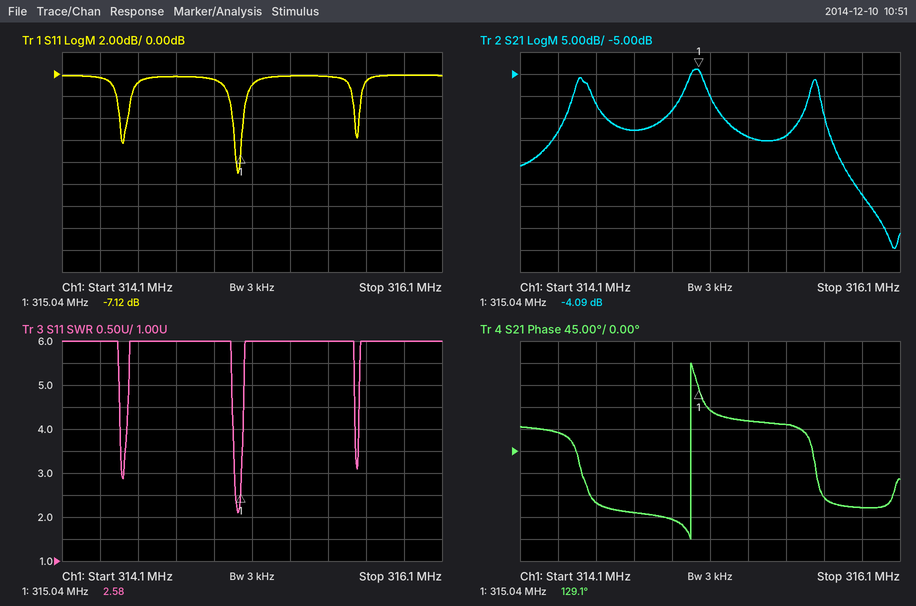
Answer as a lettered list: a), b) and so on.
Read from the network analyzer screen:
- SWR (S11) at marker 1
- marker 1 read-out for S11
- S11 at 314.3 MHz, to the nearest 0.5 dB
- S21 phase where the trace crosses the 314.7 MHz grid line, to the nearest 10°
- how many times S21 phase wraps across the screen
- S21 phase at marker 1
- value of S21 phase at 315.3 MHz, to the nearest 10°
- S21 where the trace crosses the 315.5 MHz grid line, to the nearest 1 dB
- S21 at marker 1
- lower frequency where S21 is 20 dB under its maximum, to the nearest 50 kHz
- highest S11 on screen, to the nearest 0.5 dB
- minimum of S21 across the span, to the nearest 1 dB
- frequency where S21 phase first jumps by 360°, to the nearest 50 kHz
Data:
a) 2.58
b) -7.12 dB
c) -0.5 dB
d) -130°
e) 1
f) 129.1°
g) 60°
h) -19 dB
i) -4.09 dB
j) 314.20 MHz
k) 0.0 dB
l) -45 dB
m) 315.00 MHz
